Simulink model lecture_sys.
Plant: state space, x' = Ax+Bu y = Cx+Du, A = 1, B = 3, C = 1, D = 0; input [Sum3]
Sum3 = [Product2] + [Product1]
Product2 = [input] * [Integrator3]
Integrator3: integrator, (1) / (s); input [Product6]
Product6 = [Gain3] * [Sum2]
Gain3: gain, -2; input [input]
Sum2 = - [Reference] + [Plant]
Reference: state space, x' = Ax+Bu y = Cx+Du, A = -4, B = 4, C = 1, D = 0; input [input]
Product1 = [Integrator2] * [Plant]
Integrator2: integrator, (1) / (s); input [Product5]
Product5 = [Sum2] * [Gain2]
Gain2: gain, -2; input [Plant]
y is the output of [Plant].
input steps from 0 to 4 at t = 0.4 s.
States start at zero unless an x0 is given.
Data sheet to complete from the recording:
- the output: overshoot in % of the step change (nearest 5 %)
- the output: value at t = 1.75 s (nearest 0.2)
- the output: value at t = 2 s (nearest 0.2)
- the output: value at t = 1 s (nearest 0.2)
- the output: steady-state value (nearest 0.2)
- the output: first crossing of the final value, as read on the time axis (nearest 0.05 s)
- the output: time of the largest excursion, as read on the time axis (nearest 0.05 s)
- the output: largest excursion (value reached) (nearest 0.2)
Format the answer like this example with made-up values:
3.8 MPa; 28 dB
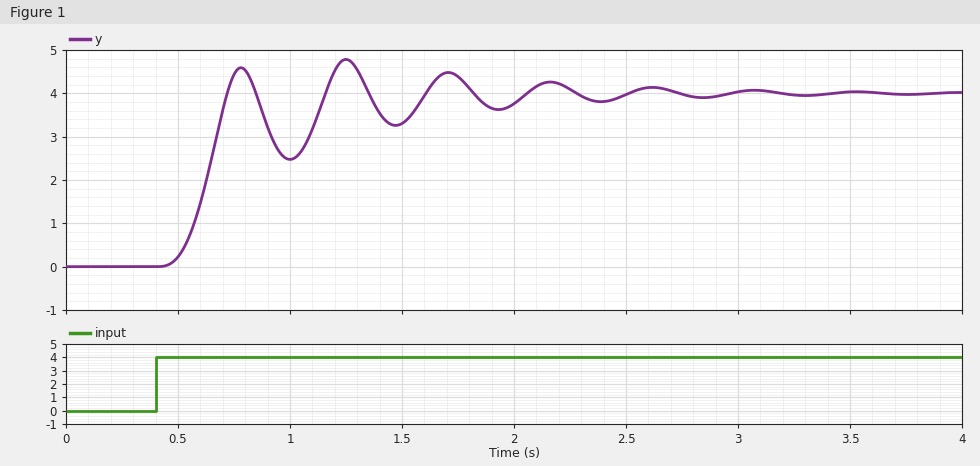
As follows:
20 %; 4.4; 3.8; 2.4; 4.0; 0.70 s; 1.25 s; 4.8
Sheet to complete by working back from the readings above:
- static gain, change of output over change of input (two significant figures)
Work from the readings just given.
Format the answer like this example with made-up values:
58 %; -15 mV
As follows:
1.0
